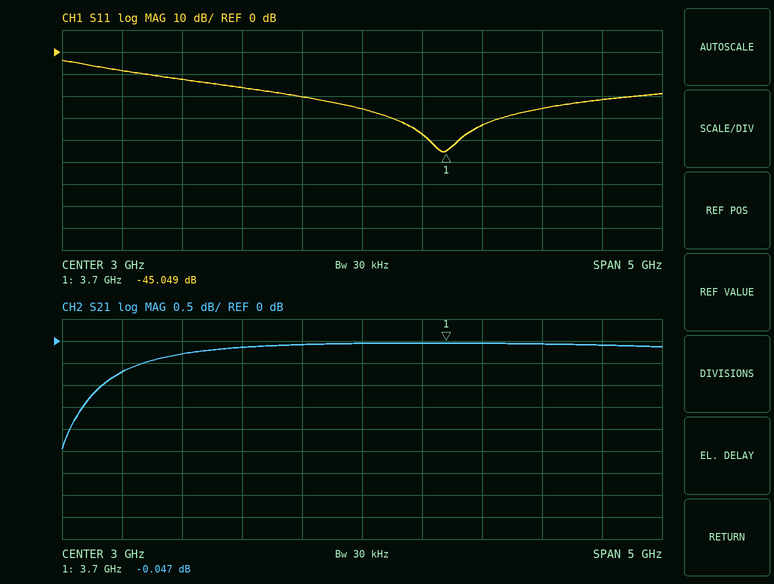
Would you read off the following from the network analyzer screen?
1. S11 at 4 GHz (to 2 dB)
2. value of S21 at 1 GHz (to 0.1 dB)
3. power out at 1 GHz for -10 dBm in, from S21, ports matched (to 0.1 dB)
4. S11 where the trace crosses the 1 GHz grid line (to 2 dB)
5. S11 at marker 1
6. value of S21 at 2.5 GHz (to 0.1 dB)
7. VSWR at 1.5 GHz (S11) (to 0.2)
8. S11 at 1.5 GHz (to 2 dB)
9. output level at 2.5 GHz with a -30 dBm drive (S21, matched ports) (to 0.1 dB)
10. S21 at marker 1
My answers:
-34 dB
-0.7 dB
-10.7 dBm
-8 dB
-45.049 dB
-0.1 dB
1.6
-12 dB
-30.1 dBm
-0.047 dB
